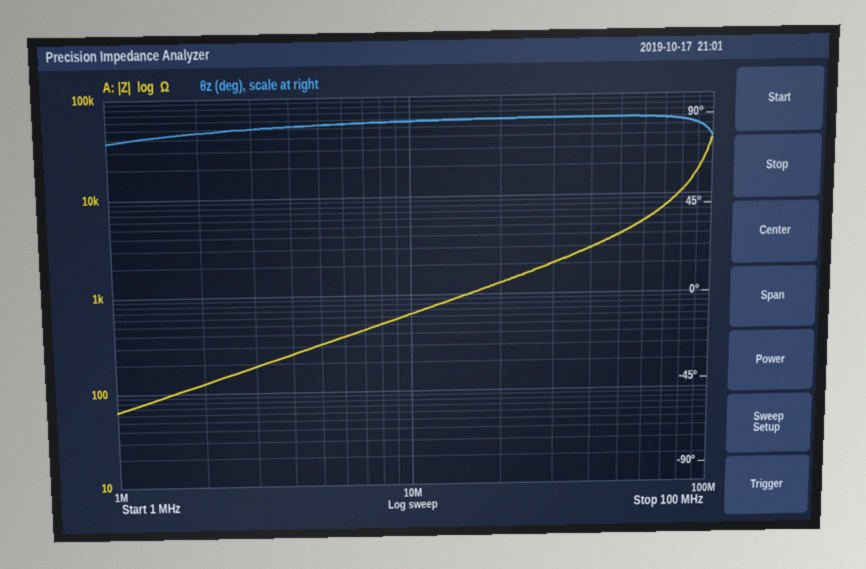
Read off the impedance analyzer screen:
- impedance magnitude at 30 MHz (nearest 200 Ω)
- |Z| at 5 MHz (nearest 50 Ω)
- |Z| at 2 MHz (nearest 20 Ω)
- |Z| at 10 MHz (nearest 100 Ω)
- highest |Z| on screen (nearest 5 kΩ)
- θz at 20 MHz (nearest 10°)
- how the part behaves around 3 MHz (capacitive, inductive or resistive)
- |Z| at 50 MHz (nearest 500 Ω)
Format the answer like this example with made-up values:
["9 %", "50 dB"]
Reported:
["2.0 kΩ", "300 Ω", "120 Ω", "600 Ω", "35 kΩ", "90°", "inductive", "4.0 kΩ"]
